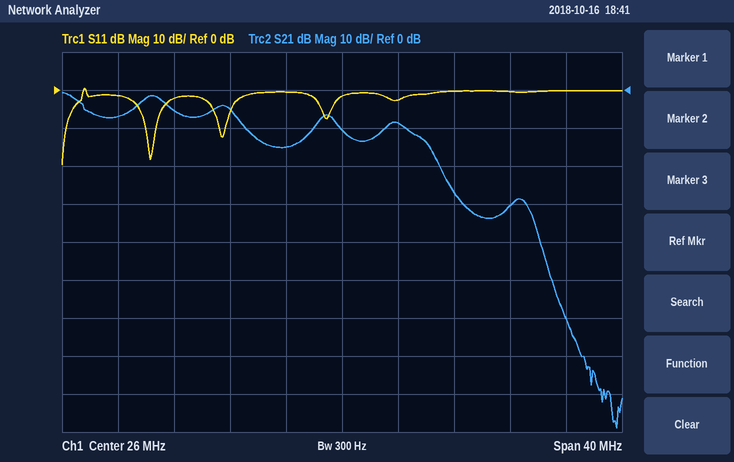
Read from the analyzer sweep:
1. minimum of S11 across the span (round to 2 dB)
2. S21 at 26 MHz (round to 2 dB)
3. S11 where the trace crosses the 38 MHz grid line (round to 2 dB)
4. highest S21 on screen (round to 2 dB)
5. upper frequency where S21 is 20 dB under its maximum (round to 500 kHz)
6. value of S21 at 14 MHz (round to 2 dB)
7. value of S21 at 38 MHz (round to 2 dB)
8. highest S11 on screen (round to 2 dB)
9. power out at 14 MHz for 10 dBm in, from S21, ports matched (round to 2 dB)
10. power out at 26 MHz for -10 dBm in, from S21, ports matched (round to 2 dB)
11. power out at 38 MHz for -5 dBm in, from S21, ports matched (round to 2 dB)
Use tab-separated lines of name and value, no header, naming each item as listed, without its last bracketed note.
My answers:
minimum of S11 across the span	-20 dB
S21 at 26 MHz	-10 dB
S11 where the trace crosses the 38 MHz grid line	0 dB
highest S21 on screen	0 dB
upper frequency where S21 is 20 dB under its maximum	33.0 MHz
value of S21 at 14 MHz	-6 dB
value of S21 at 38 MHz	-30 dB
highest S11 on screen	0 dB
power out at 14 MHz for 10 dBm in, from S21, ports matched	4 dBm
power out at 26 MHz for -10 dBm in, from S21, ports matched	-20 dBm
power out at 38 MHz for -5 dBm in, from S21, ports matched	-36 dBm
